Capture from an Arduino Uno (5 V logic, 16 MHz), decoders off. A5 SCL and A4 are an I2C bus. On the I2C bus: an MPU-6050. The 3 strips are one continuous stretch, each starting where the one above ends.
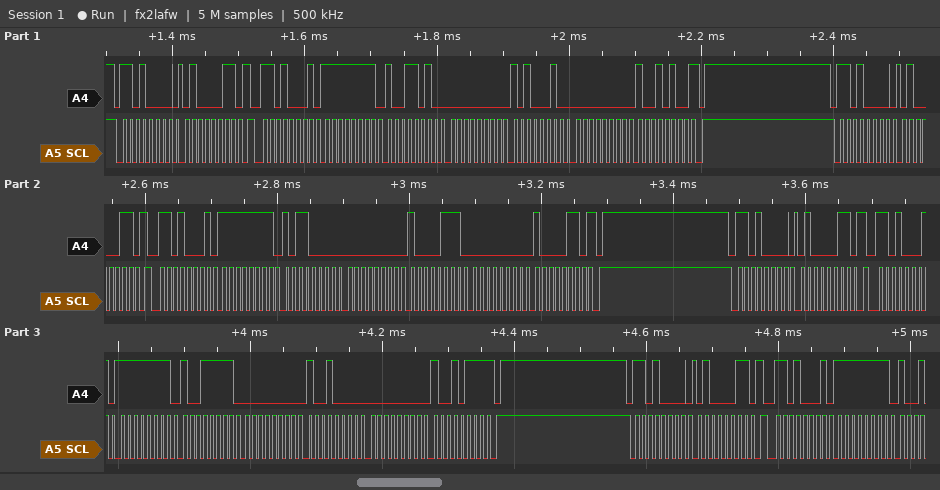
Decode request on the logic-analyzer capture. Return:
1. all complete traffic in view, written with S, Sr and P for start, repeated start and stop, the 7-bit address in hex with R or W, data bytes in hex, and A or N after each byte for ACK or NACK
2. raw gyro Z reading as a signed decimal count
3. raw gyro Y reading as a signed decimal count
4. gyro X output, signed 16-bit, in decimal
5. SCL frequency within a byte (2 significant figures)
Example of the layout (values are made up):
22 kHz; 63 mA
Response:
S 68W A 43 A Sr 68R A FF A 9A A 00 A A2 A 00 A 94 N P S 68W A 43 A Sr 68R A FF A B0 A 00 A 87 A 00 A 86 N P S 68W A 43 A Sr 68R A FF A 9F A 00 A 90 A 00 A 97 N P S 68W A 43 A Sr 68R A FF A; 148; 162; -102; 100 kHz
